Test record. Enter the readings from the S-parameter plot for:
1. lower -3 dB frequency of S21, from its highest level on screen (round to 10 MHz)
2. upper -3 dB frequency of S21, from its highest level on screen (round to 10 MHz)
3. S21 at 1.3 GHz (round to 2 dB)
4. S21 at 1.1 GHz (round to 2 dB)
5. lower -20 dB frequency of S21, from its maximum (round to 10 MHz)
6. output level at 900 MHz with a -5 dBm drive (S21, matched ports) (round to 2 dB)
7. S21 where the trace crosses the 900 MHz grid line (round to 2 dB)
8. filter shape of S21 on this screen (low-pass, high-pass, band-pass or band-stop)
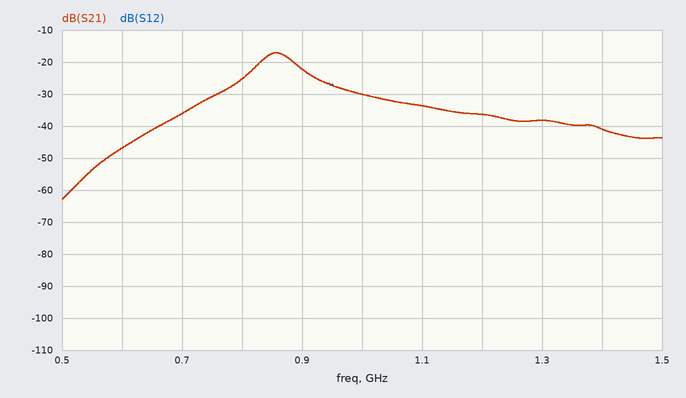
830 MHz
890 MHz
-38 dB
-34 dB
690 MHz
-28 dBm
-22 dB
band-pass
